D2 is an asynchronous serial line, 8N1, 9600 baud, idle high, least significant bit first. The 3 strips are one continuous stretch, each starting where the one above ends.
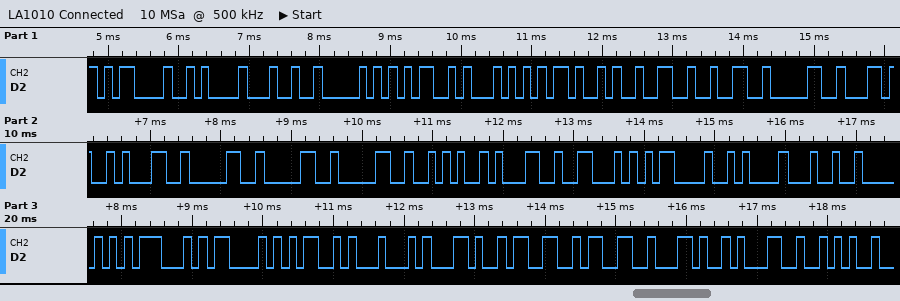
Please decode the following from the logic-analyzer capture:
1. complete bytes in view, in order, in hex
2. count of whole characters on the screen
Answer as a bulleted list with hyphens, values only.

- 0D 0A 24 50 4D 54 4B 32 32 30 2C 31 30 30 30 2A 31 46 0D 0A 24 50 47 43 4D 44 2C 33 33 2C 31 2A
- 32
